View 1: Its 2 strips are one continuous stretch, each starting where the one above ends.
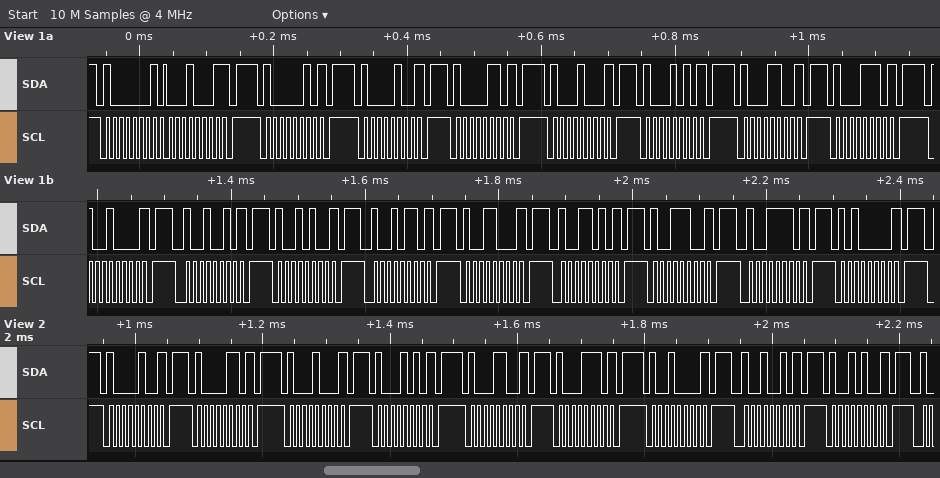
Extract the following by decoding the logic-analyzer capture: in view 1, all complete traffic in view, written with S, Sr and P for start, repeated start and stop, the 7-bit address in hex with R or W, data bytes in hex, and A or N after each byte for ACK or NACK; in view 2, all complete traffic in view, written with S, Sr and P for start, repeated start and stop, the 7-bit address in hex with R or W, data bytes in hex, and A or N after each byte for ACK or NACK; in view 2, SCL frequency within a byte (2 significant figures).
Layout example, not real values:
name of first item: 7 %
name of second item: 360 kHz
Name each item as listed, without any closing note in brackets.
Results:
in view 1, all complete traffic in view, written with S, Sr and P for start, repeated start and stop, the 7-bit address in hex with R or W, data bytes in hex, and A or N after each byte for ACK or NACK: S 40R A 11 N P S 41W N P S 42W N P S 43W N P S 44W N P S 45W N P S 46W N P S 47W N P S 48W N P S 49W N P S 4AW N P S 4BW N P S 4CW N P S 4DW N P S 4EW N P S 4FW N P S 50W N P
in view 2, all complete traffic in view, written with S, Sr and P for start, repeated start and stop, the 7-bit address in hex with R or W, data bytes in hex, and A or N after each byte for ACK or NACK: S 42W N P S 43W N P S 44W N P S 45W N P S 46W N P S 47W N P S 48W N P S 49W N P S 4AW N P
in view 2, SCL frequency within a byte: 100 kHz
